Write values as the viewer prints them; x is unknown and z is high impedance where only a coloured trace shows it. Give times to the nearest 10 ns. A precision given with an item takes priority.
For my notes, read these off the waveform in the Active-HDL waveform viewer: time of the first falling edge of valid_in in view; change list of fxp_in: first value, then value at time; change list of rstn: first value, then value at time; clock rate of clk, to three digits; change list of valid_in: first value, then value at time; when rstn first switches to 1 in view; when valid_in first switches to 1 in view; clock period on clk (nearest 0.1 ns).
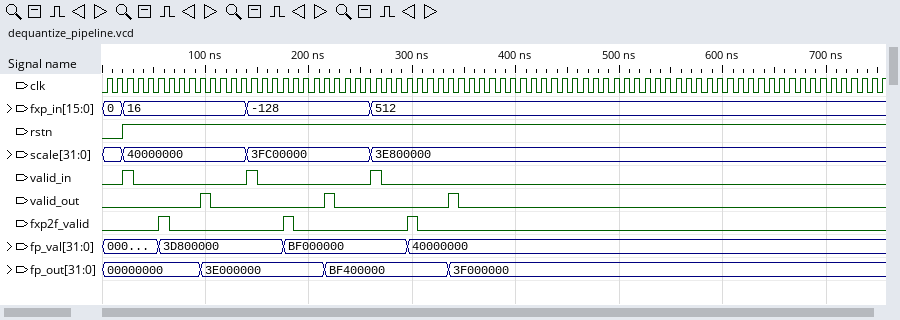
30 ns
0, 16 at 20 ns, -128 at 140 ns, 512 at 260 ns
0, 1 at 20 ns
100 MHz
0, 1 at 20 ns, 0 at 30 ns, 1 at 140 ns, 0 at 150 ns, 1 at 260 ns, 0 at 270 ns
20 ns
20 ns
10 ns
